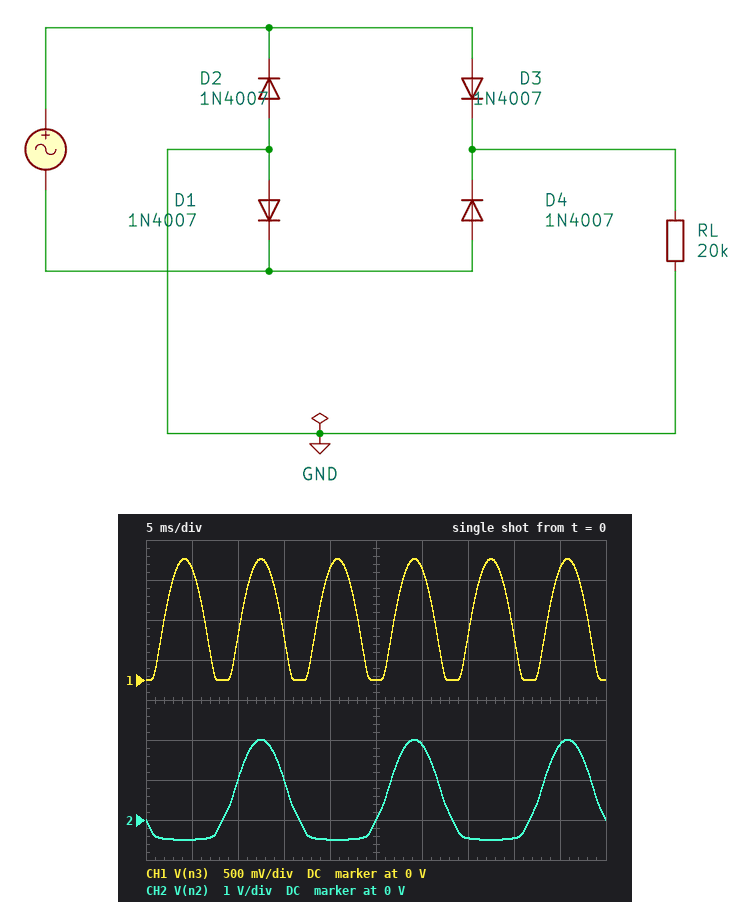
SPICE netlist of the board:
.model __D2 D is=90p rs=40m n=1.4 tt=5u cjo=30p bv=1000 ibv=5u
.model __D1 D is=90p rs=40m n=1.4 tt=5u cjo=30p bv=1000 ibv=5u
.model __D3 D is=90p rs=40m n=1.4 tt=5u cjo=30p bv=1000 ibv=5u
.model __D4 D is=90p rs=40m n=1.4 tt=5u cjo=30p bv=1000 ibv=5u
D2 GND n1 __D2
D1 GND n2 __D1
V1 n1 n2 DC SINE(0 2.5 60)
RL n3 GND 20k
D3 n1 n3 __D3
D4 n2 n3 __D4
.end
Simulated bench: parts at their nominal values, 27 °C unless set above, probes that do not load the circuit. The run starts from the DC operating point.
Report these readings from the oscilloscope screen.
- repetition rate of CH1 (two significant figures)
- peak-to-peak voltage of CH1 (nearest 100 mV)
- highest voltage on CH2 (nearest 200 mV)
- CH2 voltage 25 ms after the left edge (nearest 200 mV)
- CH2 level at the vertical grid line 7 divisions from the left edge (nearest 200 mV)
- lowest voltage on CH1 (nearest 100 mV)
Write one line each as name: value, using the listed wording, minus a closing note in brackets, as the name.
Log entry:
repetition rate of CH1: 120 Hz
peak-to-peak voltage of CH1: 1.5 V
highest voltage on CH2: 2.0 V
CH2 voltage 25 ms after the left edge: 0 V
CH2 level at the vertical grid line 7 divisions from the left edge: -400 mV
lowest voltage on CH1: 0 V
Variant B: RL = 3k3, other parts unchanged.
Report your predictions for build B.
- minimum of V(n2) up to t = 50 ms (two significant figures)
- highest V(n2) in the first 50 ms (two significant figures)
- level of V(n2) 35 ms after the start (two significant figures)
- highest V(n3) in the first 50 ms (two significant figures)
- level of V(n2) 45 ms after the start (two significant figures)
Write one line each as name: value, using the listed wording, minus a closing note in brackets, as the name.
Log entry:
minimum of V(n2) up to t = 50 ms: -560 mV
highest V(n2) in the first 50 ms: 1.9 V
level of V(n2) 35 ms after the start: -510 mV
highest V(n3) in the first 50 ms: 1.4 V
level of V(n2) 45 ms after the start: 1.8 V
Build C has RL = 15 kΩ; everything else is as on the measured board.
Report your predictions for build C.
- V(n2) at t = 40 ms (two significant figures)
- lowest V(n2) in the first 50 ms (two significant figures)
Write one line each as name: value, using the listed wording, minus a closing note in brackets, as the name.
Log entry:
V(n2) at t = 40 ms: -470 mV
lowest V(n2) in the first 50 ms: -500 mV
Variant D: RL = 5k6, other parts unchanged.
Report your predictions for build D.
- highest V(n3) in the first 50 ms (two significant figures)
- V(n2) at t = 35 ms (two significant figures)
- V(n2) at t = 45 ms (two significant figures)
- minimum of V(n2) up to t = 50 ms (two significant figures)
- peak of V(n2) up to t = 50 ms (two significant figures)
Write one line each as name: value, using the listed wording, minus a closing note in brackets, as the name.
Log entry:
highest V(n3) in the first 50 ms: 1.4 V
V(n2) at t = 35 ms: -500 mV
V(n2) at t = 45 ms: 1.8 V
minimum of V(n2) up to t = 50 ms: -540 mV
peak of V(n2) up to t = 50 ms: 2.0 V
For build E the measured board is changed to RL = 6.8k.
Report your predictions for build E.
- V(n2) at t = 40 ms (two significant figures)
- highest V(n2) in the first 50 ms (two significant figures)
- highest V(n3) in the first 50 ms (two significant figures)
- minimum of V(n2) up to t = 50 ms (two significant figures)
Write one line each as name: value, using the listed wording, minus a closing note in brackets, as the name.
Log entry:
V(n2) at t = 40 ms: -490 mV
highest V(n2) in the first 50 ms: 2.0 V
highest V(n3) in the first 50 ms: 1.4 V
minimum of V(n2) up to t = 50 ms: -530 mV
